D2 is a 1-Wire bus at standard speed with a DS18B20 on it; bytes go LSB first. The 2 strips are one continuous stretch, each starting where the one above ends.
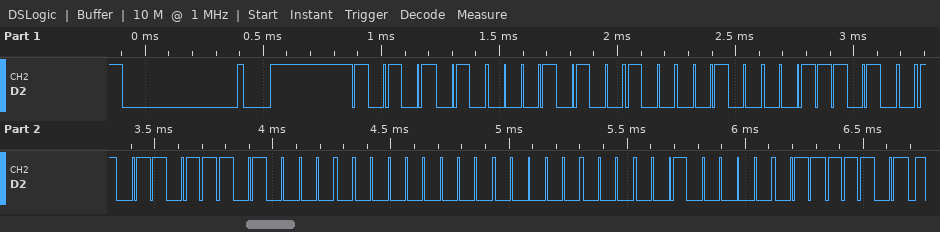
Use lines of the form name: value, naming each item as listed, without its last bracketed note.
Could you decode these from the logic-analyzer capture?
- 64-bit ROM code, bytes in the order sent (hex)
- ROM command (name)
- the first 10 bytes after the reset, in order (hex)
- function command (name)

64-bit ROM code, bytes in the order sent: 28 21 5C DA 05 00 00 04
ROM command: Match ROM
the first 10 bytes after the reset, in order: 55 28 21 5C DA 05 00 00 04 BE
function command: Read Scratchpad
